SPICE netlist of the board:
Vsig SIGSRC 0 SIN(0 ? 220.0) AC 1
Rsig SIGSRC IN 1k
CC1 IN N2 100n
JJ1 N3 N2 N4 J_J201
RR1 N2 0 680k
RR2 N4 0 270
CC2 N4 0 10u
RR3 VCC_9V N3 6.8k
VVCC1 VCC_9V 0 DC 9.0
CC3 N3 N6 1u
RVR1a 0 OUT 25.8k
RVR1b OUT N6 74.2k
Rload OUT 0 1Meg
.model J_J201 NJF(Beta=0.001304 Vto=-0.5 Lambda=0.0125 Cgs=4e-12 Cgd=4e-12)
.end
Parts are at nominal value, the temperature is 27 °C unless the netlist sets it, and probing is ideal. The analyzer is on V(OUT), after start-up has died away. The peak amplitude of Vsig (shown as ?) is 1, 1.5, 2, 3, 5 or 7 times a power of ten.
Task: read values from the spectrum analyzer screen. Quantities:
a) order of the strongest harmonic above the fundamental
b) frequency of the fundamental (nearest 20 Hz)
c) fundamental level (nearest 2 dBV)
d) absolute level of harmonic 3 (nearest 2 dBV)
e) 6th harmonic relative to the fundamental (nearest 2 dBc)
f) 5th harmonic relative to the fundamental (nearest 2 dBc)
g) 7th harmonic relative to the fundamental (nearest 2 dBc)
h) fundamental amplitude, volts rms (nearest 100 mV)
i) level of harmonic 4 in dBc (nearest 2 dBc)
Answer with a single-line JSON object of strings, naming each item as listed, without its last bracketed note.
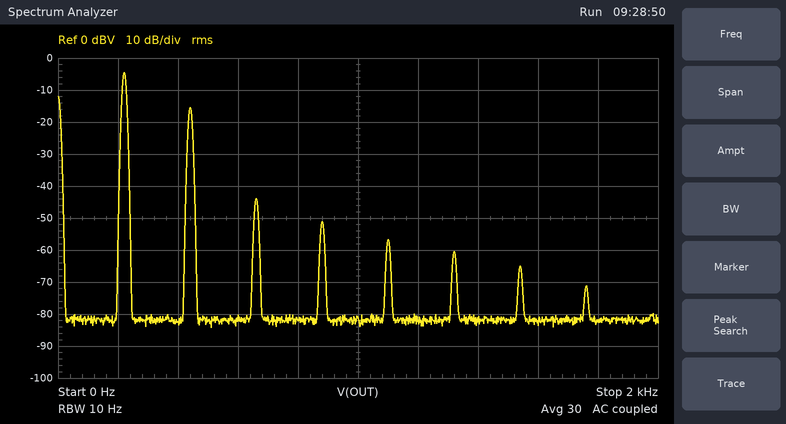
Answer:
{"order of the strongest harmonic above the fundamental": "2", "frequency of the fundamental": "220 Hz", "fundamental level": "-4 dBV", "absolute level of harmonic 3": "-44 dBV", "6th harmonic relative to the fundamental": "-56 dBc", "5th harmonic relative to the fundamental": "-52 dBc", "7th harmonic relative to the fundamental": "-60 dBc", "fundamental amplitude, volts rms": "600 mV", "level of harmonic 4 in dBc": "-46 dBc"}
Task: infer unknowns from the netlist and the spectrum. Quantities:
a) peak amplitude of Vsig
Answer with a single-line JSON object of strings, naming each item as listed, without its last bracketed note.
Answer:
{"peak amplitude of Vsig": "500 mV"}
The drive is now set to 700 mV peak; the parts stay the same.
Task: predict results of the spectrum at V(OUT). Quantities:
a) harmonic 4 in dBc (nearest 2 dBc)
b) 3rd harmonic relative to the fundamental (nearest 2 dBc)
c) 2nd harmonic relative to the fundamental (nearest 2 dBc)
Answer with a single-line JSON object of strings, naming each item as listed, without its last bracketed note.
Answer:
{"harmonic 4 in dBc": "-28 dBc", "3rd harmonic relative to the fundamental": "-32 dBc", "2nd harmonic relative to the fundamental": "-8 dBc"}
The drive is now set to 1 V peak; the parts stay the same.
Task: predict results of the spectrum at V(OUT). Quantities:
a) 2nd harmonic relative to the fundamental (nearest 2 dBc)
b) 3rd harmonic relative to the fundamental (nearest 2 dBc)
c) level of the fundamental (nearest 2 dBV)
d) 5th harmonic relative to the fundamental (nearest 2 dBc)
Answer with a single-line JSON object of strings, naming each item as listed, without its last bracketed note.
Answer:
{"2nd harmonic relative to the fundamental": "-6 dBc", "3rd harmonic relative to the fundamental": "-18 dBc", "level of the fundamental": "-4 dBV", "5th harmonic relative to the fundamental": "-26 dBc"}
